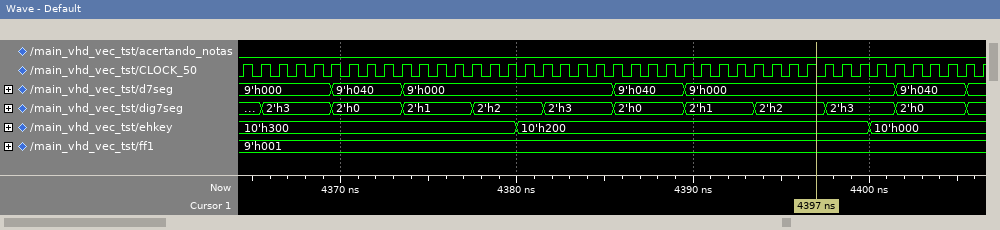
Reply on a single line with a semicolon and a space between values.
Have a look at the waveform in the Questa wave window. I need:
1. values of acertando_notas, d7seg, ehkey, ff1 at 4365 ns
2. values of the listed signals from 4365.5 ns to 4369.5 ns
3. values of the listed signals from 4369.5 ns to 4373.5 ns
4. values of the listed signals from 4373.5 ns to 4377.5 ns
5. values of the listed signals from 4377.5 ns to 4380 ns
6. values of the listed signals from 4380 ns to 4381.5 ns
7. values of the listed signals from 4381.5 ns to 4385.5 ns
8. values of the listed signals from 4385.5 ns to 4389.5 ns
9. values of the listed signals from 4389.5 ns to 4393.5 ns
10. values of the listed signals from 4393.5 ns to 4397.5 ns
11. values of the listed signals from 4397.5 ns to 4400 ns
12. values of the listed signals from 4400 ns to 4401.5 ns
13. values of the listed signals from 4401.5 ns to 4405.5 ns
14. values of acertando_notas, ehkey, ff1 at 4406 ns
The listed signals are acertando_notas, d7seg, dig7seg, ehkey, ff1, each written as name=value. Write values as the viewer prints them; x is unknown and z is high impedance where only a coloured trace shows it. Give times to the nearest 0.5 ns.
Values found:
acertando_notas=0, d7seg=9'h000, ehkey=10'h300, ff1=9'h001; acertando_notas=0, d7seg=9'h000, dig7seg=2'h3, ehkey=10'h300, ff1=9'h001; acertando_notas=0, d7seg=9'h040, dig7seg=2'h0, ehkey=10'h300, ff1=9'h001; acertando_notas=0, d7seg=9'h000, dig7seg=2'h1, ehkey=10'h300, ff1=9'h001; acertando_notas=0, d7seg=9'h000, dig7seg=2'h2, ehkey=10'h300, ff1=9'h001; acertando_notas=0, d7seg=9'h000, dig7seg=2'h2, ehkey=10'h200, ff1=9'h001; acertando_notas=0, d7seg=9'h000, dig7seg=2'h3, ehkey=10'h200, ff1=9'h001; acertando_notas=0, d7seg=9'h040, dig7seg=2'h0, ehkey=10'h200, ff1=9'h001; acertando_notas=0, d7seg=9'h000, dig7seg=2'h1, ehkey=10'h200, ff1=9'h001; acertando_notas=0, d7seg=9'h000, dig7seg=2'h2, ehkey=10'h200, ff1=9'h001; acertando_notas=0, d7seg=9'h000, dig7seg=2'h3, ehkey=10'h200, ff1=9'h001; acertando_notas=0, d7seg=9'h000, dig7seg=2'h3, ehkey=10'h000, ff1=9'h001; acertando_notas=0, d7seg=9'h040, dig7seg=2'h0, ehkey=10'h000, ff1=9'h001; acertando_notas=0, ehkey=10'h000, ff1=9'h001
